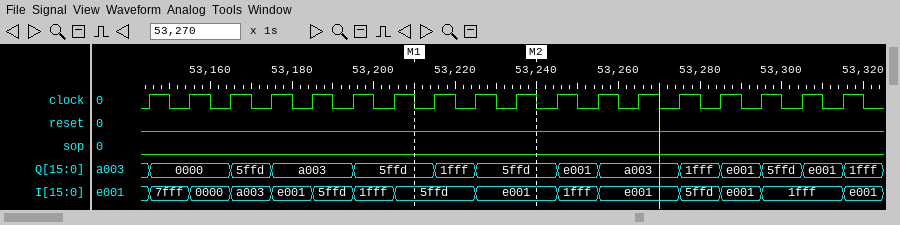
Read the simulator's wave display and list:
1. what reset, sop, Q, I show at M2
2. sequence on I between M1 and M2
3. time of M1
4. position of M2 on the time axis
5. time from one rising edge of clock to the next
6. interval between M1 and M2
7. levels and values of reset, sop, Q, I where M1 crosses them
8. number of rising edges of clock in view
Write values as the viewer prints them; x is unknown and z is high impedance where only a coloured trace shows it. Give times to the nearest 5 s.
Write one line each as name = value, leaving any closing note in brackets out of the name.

what reset, sop, Q, I show at M2 = reset=0, sop=0, Q=5ffd, I=e001
sequence on I between M1 and M2 = 5ffd, e001
time of M1 = 53210 s
position of M2 on the time axis = 53240 s
time from one rising edge of clock to the next = 10 s
interval between M1 and M2 = 30 s
levels and values of reset, sop, Q, I where M1 crosses them = reset=0, sop=0, Q=5ffd, I=5ffd
number of rising edges of clock in view = 18
